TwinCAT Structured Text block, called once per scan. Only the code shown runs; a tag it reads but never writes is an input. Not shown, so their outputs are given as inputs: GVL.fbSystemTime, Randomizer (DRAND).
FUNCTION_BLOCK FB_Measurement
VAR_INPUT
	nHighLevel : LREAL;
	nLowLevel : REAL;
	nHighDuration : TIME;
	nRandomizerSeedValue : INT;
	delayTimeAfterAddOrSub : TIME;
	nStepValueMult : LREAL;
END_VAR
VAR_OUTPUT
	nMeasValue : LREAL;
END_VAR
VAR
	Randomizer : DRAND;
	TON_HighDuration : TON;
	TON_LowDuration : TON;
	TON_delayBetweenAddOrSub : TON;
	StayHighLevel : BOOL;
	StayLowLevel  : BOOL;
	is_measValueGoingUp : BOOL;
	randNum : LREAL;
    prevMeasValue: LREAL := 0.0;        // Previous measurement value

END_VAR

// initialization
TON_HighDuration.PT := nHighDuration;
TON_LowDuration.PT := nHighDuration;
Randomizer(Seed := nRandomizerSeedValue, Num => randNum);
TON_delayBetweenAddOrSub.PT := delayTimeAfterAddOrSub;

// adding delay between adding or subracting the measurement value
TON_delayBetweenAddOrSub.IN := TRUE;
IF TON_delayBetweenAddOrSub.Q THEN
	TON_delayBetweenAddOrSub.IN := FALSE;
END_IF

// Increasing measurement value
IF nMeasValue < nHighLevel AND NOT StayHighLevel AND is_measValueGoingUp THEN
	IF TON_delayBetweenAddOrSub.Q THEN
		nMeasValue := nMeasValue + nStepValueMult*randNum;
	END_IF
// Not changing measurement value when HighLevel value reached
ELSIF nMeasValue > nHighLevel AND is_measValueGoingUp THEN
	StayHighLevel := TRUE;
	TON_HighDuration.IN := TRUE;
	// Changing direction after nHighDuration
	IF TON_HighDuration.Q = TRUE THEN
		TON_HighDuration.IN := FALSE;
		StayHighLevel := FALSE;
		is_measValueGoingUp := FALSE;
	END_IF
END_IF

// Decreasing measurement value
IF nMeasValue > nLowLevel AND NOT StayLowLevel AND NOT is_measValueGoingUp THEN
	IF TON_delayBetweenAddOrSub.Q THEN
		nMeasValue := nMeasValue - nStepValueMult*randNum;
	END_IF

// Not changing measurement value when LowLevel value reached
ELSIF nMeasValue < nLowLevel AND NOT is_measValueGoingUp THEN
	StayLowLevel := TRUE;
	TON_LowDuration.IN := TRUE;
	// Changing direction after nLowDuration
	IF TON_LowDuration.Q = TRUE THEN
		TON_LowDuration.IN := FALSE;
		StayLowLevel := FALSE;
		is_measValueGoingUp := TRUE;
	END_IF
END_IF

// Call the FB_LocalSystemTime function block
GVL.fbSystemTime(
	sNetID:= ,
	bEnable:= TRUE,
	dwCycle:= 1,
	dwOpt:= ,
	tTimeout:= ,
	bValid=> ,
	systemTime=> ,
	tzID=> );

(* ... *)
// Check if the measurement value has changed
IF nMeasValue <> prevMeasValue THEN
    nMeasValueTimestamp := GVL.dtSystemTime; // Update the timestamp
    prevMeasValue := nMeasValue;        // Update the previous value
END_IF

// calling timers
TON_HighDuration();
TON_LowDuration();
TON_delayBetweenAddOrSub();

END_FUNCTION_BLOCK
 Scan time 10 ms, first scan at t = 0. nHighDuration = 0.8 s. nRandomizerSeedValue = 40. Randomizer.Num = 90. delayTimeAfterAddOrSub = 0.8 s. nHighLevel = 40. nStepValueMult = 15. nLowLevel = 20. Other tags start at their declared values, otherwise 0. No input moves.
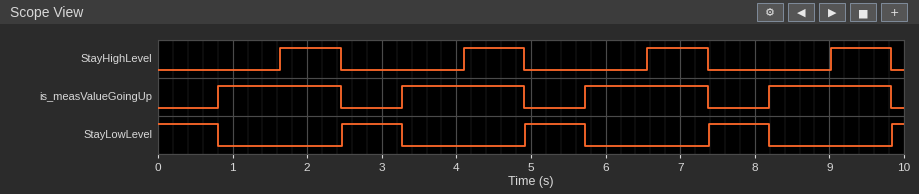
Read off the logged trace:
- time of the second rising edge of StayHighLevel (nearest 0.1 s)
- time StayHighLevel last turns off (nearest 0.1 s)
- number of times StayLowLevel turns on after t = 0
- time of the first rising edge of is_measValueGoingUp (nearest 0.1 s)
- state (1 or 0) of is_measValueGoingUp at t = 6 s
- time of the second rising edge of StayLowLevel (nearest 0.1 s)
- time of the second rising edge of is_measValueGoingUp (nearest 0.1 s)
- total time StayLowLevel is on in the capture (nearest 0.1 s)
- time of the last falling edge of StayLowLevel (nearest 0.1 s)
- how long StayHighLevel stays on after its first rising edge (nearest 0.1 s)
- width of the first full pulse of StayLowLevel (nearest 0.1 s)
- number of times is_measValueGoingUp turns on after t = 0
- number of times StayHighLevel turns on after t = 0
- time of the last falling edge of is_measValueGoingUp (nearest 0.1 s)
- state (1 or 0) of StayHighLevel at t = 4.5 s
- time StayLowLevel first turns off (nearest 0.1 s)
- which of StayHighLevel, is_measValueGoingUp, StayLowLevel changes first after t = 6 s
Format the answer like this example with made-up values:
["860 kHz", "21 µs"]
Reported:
["4.1 s", "9.8 s", "4", "0.8 s", "1", "4.9 s", "3.3 s", "3.4 s", "8.2 s", "0.8 s", "0.8 s", "4", "4", "9.8 s", "1", "0.8 s", "StayHighLevel"]
